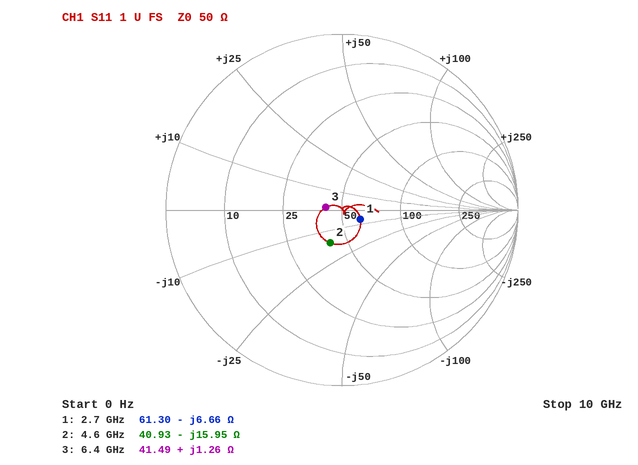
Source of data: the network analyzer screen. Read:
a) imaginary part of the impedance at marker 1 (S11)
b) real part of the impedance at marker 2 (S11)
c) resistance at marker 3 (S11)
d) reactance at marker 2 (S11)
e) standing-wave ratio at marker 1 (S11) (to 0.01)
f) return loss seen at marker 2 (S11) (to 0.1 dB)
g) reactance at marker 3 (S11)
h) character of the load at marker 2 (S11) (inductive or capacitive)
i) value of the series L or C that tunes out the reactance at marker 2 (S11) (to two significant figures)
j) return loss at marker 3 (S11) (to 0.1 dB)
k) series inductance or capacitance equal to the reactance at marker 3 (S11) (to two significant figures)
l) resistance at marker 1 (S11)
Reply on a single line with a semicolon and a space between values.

-6.66 Ω; 40.93 Ω; 41.49 Ω; -15.95 Ω; 1.27; 14.0 dB; +1.26 Ω; capacitive; 550 pH; 20.5 dB; 31 pH; 61.30 Ω
